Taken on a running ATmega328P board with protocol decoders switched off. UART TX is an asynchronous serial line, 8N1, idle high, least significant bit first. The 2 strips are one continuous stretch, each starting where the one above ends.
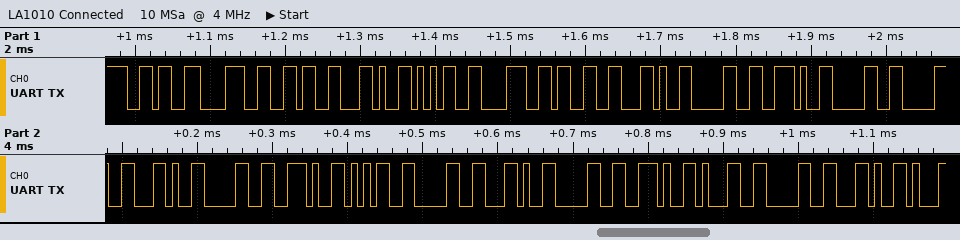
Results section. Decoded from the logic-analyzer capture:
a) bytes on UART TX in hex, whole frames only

36 38 36 2C 35 38 33 2C 30 2E 30 30 2C 30 2E 35 30 2C 30 2E 31 30 2C
